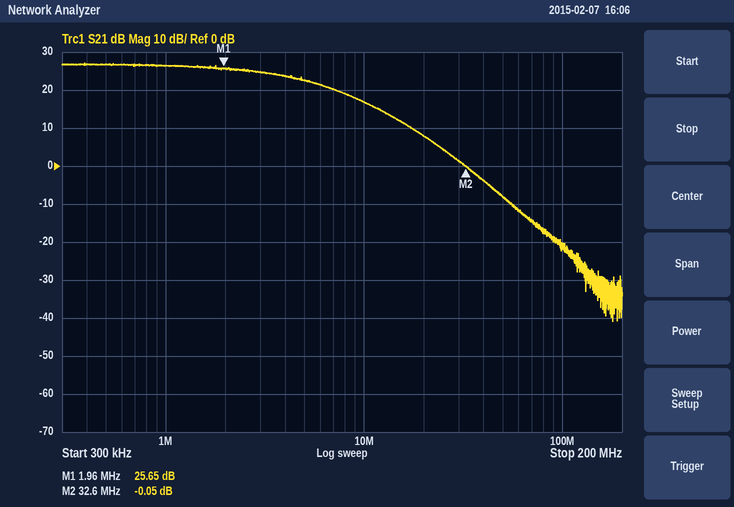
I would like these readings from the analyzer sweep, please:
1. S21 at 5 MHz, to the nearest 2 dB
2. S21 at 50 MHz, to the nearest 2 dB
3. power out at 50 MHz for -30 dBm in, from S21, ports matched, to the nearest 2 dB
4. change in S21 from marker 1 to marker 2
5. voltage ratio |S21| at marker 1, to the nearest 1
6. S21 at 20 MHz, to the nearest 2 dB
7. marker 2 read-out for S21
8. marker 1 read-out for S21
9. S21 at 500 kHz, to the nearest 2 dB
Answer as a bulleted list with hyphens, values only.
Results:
- 22 dB
- -8 dB
- -38 dBm
- -25.70 dB
- 19
- 8 dB
- -0.05 dB
- 25.65 dB
- 26 dB
